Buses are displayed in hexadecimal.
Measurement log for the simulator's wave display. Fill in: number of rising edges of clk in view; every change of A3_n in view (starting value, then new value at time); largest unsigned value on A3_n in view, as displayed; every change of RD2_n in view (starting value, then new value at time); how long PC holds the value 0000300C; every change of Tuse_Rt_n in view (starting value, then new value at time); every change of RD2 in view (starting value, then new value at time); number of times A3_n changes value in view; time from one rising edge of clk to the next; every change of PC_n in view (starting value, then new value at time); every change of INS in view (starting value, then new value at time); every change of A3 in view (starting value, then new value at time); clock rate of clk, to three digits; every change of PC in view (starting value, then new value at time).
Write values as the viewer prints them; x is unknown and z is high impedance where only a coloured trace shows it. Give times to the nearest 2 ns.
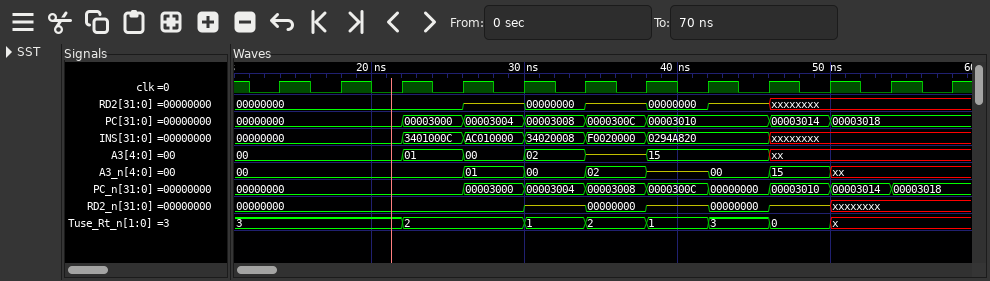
12
00, 01 at 26 ns, 00 at 30 ns, 02 at 34 ns, z at 38 ns, 00 at 42 ns, 15 at 46 ns, xx at 50 ns
15
00000000, z at 30 ns, 00000000 at 34 ns, z at 38 ns, 00000000 at 42 ns, z at 46 ns, xxxxxxxx at 50 ns
4 ns
3, 2 at 22 ns, 1 at 30 ns, 2 at 34 ns, 1 at 38 ns, 3 at 42 ns, 0 at 46 ns, x at 50 ns
00000000, z at 26 ns, 00000000 at 30 ns, z at 34 ns, 00000000 at 38 ns, z at 42 ns, xxxxxxxx at 46 ns
7
4 ns
00000000, 00003000 at 26 ns, 00003004 at 30 ns, 00003008 at 34 ns, 0000300C at 38 ns, 00000000 at 42 ns, 00003010 at 46 ns, 00003014 at 50 ns, 00003018 at 54 ns
00000000, 3401000C at 22 ns, AC010000 at 26 ns, 34020008 at 30 ns, F0020000 at 34 ns, 0294A820 at 38 ns, xxxxxxxx at 46 ns
00, 01 at 22 ns, 00 at 26 ns, 02 at 30 ns, z at 34 ns, 15 at 38 ns, xx at 46 ns
250 MHz
00000000, 00003000 at 22 ns, 00003004 at 26 ns, 00003008 at 30 ns, 0000300C at 34 ns, 00003010 at 38 ns, 00003014 at 46 ns, 00003018 at 50 ns
